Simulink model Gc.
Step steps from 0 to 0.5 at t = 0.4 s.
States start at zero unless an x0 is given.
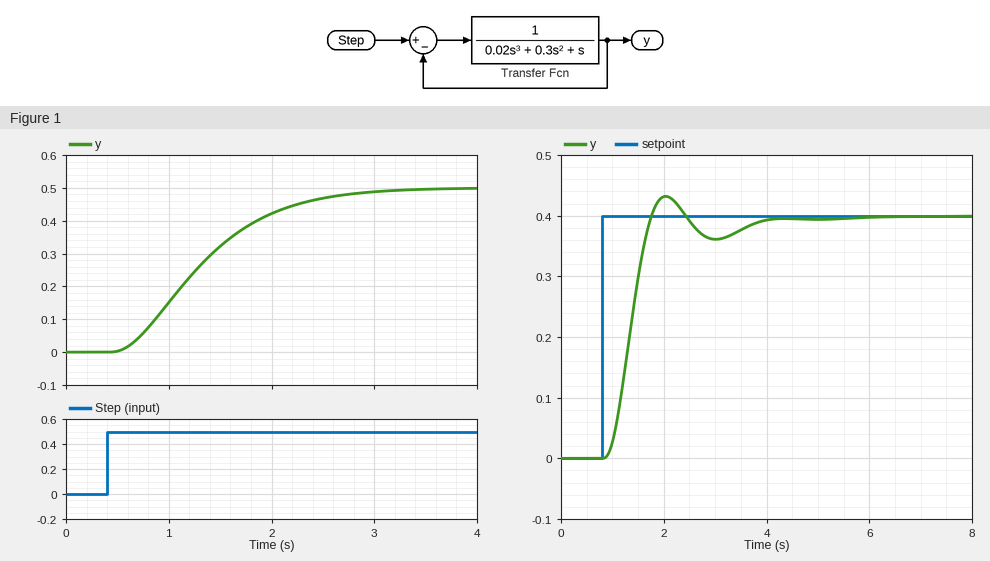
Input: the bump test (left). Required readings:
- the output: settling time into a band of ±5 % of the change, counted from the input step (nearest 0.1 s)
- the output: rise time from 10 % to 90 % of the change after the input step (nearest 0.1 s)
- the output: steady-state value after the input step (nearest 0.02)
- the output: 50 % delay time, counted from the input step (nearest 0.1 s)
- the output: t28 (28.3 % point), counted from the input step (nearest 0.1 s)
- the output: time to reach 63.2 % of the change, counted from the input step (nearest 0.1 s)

2.2 s
1.5 s
0.50
0.9 s
0.6 s
1.1 s
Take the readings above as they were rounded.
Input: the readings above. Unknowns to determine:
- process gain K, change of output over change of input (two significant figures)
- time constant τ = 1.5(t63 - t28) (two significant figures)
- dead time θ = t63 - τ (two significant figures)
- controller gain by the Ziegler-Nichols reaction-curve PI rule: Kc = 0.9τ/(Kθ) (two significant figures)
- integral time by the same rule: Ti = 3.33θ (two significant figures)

1.0
0.75 s
0.35 s
1.9
1.2 s
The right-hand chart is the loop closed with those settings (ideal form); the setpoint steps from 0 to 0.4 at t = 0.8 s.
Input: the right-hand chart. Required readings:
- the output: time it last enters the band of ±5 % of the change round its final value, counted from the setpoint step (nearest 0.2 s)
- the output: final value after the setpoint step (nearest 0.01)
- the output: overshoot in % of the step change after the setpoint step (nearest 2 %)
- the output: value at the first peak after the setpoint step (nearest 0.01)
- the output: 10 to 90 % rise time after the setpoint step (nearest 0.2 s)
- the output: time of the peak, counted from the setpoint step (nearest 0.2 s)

2.8 s
0.40
8 %
0.43
0.6 s
1.2 s
